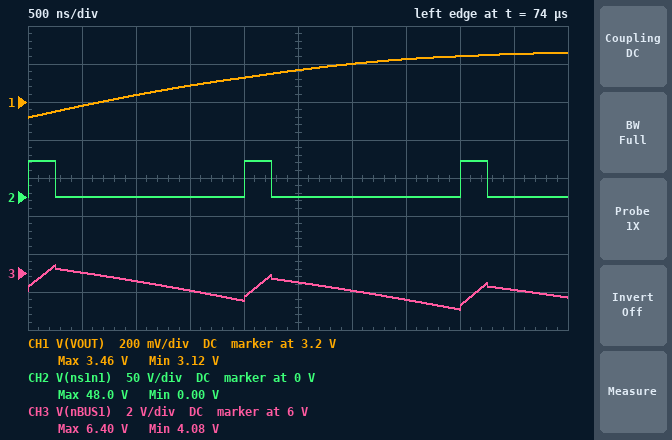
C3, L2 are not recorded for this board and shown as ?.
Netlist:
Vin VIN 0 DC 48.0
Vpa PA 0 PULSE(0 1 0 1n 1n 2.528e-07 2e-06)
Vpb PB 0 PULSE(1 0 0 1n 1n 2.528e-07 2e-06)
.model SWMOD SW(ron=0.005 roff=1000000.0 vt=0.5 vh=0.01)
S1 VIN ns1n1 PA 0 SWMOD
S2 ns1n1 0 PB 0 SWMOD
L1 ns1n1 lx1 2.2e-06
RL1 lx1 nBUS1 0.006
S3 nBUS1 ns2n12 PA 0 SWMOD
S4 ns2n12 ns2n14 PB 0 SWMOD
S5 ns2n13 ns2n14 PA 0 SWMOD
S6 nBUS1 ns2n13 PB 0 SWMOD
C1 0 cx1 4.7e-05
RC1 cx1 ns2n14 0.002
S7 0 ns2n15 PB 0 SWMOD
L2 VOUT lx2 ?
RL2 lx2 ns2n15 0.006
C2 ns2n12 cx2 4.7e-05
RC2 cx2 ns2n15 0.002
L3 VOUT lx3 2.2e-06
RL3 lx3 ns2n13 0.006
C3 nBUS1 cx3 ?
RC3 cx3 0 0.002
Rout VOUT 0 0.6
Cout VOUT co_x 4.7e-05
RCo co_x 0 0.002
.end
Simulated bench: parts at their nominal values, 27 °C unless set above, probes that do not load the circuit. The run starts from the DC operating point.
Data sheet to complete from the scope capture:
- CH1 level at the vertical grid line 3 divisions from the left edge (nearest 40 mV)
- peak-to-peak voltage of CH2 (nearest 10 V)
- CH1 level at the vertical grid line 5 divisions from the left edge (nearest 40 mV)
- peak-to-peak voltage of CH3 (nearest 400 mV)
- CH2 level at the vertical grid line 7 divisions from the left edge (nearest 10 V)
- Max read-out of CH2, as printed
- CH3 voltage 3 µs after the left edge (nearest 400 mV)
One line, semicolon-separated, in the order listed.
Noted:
3.28 V; 50 V; 3.36 V; 2.4 V; 0 V; 48.0 V; 5.2 V
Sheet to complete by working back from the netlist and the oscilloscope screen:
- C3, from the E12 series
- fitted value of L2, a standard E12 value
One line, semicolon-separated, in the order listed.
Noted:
18 µF; 1.5 µH
